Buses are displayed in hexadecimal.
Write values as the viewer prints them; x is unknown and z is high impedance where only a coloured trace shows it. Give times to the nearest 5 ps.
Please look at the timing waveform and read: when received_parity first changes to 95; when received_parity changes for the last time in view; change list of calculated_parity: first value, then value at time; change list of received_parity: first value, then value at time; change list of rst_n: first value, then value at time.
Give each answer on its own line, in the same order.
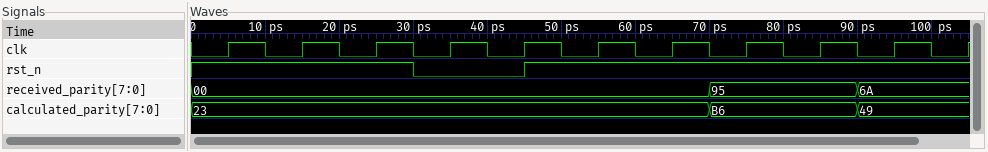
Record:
70 ps
90 ps
23, B6 at 70 ps, 49 at 90 ps
00, 95 at 70 ps, 6A at 90 ps
1, 0 at 30 ps, 1 at 45 ps
